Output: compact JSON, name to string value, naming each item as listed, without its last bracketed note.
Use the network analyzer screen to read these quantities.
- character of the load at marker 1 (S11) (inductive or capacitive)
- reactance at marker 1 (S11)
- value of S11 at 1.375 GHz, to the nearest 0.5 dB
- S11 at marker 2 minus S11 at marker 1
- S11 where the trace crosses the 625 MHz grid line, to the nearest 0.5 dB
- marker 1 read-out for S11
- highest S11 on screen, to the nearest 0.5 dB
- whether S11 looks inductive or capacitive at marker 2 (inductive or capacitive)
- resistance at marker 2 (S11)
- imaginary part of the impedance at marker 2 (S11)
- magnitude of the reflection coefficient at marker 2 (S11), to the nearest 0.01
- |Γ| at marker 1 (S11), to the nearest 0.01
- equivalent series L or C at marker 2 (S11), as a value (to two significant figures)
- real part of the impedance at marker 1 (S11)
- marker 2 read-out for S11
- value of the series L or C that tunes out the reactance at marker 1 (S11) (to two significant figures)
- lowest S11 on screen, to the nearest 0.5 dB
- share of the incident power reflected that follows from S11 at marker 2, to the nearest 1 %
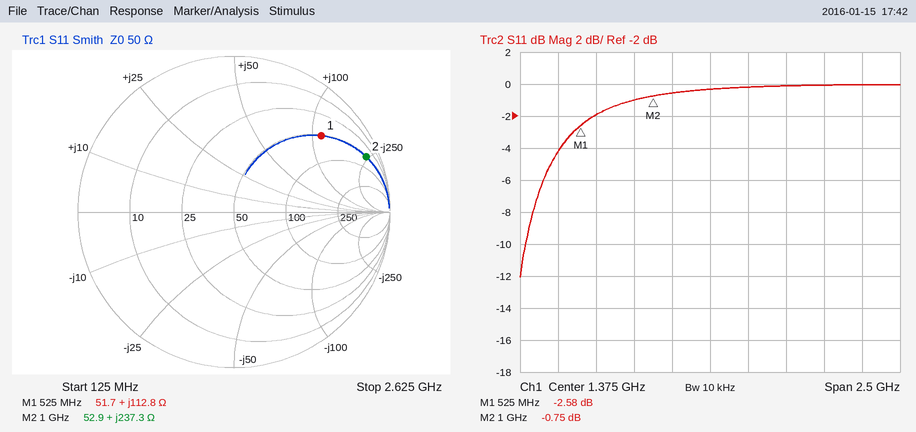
{"character of the load at marker 1 (S11)": "inductive", "reactance at marker 1": "+112.8 Ω", "value of S11 at 1.375 GHz, to the nearest 0.5 dB": "-0.5 dB", "S11 at marker 2 minus S11 at marker 1": "1.83 dB", "S11 where the trace crosses the 625 MHz grid line, to the nearest 0.5 dB": "-2.0 dB", "marker 1 read-out for S11": "-2.58 dB", "highest S11 on screen, to the nearest 0.5 dB": "0.0 dB", "whether S11 looks inductive or capacitive at marker 2": "inductive", "resistance at marker 2": "52.9 Ω", "imaginary part of the impedance at marker 2": "+237.3 Ω", "magnitude of the reflection coefficient at marker 2 (S11), to the nearest 0.01": "0.92", "|Γ| at marker 1 (S11), to the nearest 0.01": "0.74", "equivalent series L or C at marker 2 (S11), as a value": "38 nH", "real part of the impedance at marker 1": "51.7 Ω", "marker 2 read-out for S11": "-0.75 dB", "value of the series L or C that tunes out the reactance at marker 1 (S11)": "2.7 pF", "lowest S11 on screen, to the nearest 0.5 dB": "-12.0 dB", "share of the incident power reflected that follows from S11 at marker 2, to the nearest 1 %": "84 %"}
